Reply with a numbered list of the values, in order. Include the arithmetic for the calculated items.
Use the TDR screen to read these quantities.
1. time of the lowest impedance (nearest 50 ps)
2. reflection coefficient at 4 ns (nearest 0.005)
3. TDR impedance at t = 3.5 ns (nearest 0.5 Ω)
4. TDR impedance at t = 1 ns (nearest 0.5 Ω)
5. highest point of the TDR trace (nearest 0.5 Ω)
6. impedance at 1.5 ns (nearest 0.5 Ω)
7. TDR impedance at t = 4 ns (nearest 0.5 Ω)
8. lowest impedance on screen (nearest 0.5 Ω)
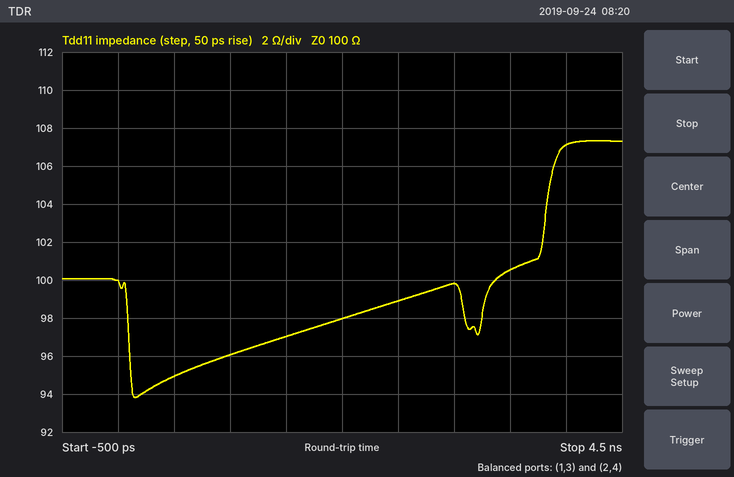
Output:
1. 150 ps
2. (107 − 100)/(107 + 100) ≈ +0.0338, so +0.035 to the nearest 0.005
3. 100.5 Ω
4. 96.0 Ω
5. 107.5 Ω
6. 97.0 Ω
7. 107.0 Ω
8. 94.0 Ω
